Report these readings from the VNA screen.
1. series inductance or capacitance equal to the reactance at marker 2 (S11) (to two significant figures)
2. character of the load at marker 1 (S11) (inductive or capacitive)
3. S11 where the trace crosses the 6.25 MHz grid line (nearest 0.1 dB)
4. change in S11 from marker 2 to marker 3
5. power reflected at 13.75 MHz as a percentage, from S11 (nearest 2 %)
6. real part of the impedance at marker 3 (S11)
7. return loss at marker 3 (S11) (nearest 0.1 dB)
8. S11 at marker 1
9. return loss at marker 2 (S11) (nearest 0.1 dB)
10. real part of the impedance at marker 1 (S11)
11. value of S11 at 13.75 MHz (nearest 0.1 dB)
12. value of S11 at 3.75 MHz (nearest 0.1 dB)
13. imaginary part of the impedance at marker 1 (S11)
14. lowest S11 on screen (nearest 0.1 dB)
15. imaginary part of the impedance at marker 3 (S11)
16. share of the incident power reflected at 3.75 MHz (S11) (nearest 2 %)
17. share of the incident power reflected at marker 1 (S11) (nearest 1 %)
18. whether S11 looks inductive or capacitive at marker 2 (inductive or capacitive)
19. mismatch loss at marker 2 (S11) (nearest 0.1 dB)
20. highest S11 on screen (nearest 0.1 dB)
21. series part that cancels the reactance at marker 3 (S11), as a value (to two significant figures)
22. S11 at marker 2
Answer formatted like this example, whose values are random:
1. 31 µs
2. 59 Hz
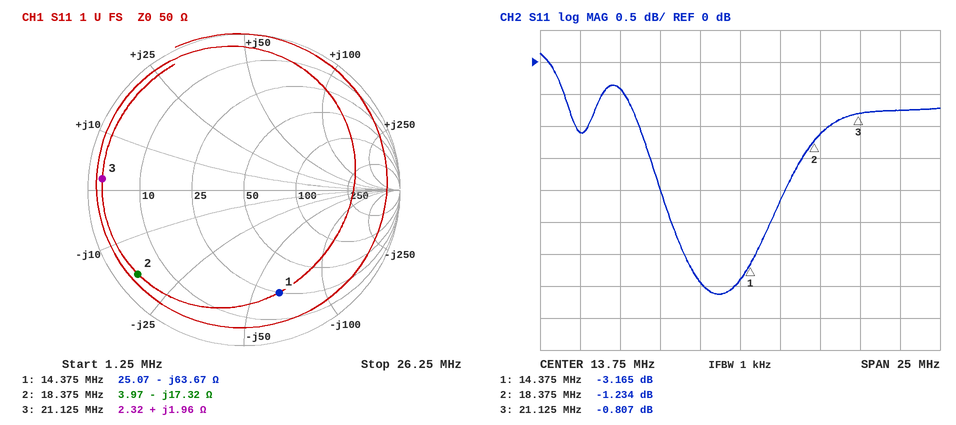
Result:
1. 500 pF
2. capacitive
3. -0.4 dB
4. 0.427 dB
5. 46 %
6. 2.32 Ω
7. 0.8 dB
8. -3.165 dB
9. 1.2 dB
10. 25.07 Ω
11. -3.4 dB
12. -1.1 dB
13. -63.67 Ω
14. -3.6 dB
15. +1.96 Ω
16. 78 %
17. 48 %
18. capacitive
19. 6.1 dB
20. 0.1 dB
21. 3.8 nF
22. -1.234 dB
